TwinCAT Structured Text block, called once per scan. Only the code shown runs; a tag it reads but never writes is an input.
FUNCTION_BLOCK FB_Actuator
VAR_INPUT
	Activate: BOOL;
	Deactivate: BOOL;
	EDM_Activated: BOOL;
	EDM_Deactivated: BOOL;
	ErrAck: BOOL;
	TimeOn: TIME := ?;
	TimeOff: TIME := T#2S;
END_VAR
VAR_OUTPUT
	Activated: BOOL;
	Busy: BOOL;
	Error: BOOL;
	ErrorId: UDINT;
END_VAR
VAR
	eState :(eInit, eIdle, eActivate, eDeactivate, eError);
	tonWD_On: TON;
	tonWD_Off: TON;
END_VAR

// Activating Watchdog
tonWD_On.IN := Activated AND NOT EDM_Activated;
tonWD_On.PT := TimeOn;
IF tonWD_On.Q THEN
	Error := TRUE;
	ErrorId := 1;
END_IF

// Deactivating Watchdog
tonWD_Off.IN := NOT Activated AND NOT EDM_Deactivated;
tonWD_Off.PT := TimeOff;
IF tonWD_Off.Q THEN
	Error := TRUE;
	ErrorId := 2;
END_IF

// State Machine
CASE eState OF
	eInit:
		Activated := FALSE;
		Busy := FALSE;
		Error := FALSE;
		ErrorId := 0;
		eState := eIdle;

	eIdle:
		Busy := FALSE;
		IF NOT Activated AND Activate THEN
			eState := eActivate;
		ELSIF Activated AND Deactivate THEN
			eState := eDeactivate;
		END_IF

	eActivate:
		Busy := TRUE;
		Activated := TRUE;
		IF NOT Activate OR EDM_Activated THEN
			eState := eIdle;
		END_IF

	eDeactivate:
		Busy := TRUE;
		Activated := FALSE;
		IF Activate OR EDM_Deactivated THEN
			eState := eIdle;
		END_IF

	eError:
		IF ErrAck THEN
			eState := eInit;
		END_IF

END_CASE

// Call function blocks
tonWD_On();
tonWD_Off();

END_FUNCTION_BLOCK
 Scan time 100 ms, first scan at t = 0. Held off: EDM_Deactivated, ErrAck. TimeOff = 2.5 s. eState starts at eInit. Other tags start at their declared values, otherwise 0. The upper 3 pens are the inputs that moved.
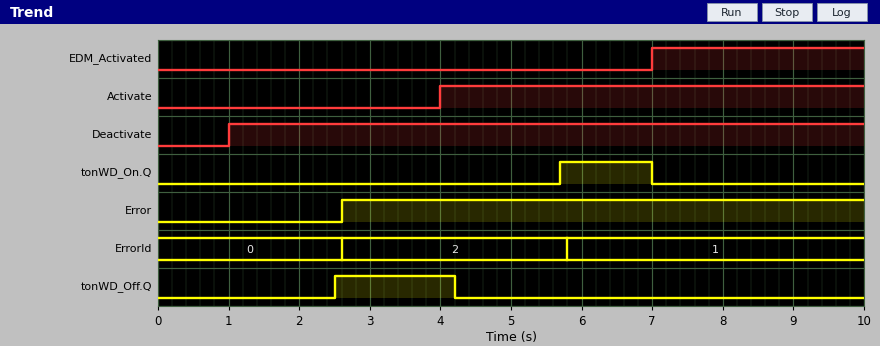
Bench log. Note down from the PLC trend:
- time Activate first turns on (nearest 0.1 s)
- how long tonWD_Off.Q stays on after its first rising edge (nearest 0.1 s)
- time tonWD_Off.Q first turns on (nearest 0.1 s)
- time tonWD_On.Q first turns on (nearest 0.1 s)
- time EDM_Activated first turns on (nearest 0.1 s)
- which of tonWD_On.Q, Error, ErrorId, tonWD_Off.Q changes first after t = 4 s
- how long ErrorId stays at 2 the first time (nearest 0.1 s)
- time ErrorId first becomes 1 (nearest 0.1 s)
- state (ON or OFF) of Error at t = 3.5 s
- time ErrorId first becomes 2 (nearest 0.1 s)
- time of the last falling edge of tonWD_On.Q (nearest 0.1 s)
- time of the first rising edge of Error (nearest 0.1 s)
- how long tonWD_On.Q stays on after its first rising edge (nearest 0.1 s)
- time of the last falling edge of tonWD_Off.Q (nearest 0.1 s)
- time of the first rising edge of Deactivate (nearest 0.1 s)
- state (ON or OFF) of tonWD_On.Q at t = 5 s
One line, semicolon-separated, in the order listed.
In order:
4.0 s; 1.7 s; 2.5 s; 5.7 s; 7.0 s; tonWD_Off.Q; 3.2 s; 5.8 s; ON; 2.6 s; 7.0 s; 2.6 s; 1.3 s; 4.2 s; 1.0 s; OFF
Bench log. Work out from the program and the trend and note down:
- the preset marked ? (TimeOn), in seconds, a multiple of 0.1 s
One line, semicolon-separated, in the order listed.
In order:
1.5 s
